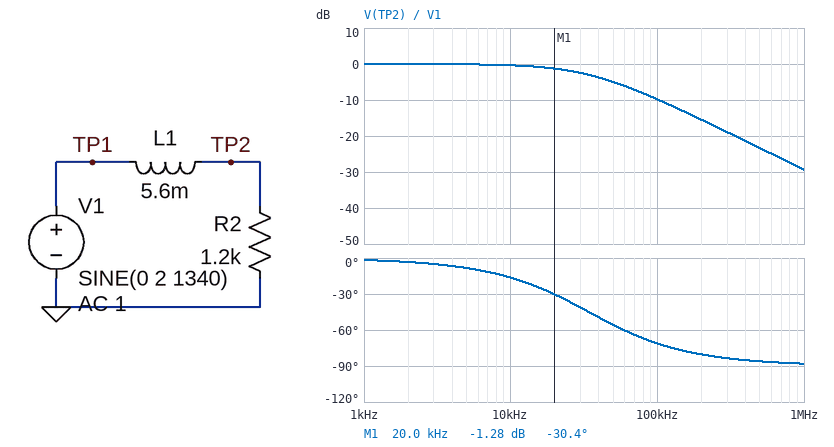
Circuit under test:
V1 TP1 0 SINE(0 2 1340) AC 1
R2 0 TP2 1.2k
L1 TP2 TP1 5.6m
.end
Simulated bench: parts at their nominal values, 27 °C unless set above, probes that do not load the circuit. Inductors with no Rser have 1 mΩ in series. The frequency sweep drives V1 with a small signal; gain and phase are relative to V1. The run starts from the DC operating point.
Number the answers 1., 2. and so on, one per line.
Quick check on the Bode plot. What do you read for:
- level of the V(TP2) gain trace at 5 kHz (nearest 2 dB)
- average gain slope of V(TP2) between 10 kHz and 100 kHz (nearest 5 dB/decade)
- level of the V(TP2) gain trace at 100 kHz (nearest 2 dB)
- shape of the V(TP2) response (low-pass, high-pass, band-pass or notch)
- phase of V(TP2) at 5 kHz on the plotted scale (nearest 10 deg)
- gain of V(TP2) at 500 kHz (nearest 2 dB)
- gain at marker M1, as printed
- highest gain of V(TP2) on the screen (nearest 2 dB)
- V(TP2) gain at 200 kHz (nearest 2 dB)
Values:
1. 0 dB
2. -10 dB/decade
3. -10 dB
4. low-pass
5. -10 deg
6. -24 dB
7. -1.28 dB
8. 0 dB
9. -16 dB
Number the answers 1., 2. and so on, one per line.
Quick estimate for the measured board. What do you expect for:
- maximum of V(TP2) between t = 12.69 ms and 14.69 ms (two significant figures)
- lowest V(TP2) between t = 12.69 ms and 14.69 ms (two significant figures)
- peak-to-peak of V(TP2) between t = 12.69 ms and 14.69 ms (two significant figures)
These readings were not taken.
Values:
1. 2.0 V
2. -2.0 V
3. 4.0 V
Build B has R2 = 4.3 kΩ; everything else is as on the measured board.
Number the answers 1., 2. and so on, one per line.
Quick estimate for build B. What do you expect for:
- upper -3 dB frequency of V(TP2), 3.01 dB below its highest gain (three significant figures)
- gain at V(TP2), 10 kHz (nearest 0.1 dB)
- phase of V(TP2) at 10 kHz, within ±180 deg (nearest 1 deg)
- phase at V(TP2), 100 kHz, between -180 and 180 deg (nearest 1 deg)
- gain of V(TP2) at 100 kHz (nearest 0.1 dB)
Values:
1. 122 kHz
2. 0 dB
3. -5 deg
4. -39 deg
5. -2.2 dB
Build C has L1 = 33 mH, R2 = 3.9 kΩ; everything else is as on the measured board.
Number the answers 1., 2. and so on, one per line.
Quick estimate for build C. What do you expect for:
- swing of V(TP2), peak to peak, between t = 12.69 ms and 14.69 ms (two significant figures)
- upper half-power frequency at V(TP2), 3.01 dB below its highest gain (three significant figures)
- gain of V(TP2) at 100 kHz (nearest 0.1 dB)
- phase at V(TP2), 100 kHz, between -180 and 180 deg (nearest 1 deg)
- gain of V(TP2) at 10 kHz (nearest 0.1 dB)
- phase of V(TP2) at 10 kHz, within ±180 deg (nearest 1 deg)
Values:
1. 4.0 V
2. 18.8 kHz
3. -14.7 dB
4. -79 deg
5. -1.1 dB
6. -28 deg
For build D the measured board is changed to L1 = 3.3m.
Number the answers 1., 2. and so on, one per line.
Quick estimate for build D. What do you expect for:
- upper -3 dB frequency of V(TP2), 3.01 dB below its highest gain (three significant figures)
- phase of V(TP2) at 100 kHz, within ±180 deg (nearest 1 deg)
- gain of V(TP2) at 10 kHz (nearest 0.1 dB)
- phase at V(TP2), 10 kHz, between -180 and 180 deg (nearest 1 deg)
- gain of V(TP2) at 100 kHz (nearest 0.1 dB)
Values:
1. 57.9 kHz
2. -60 deg
3. -0.1 dB
4. -10 deg
5. -6.0 dB
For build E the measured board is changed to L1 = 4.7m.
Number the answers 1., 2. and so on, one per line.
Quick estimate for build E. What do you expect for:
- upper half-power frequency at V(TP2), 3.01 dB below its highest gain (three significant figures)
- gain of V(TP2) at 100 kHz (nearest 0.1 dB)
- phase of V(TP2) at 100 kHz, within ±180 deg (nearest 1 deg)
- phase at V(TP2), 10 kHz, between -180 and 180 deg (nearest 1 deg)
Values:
1. 40.6 kHz
2. -8.5 dB
3. -68 deg
4. -14 deg
